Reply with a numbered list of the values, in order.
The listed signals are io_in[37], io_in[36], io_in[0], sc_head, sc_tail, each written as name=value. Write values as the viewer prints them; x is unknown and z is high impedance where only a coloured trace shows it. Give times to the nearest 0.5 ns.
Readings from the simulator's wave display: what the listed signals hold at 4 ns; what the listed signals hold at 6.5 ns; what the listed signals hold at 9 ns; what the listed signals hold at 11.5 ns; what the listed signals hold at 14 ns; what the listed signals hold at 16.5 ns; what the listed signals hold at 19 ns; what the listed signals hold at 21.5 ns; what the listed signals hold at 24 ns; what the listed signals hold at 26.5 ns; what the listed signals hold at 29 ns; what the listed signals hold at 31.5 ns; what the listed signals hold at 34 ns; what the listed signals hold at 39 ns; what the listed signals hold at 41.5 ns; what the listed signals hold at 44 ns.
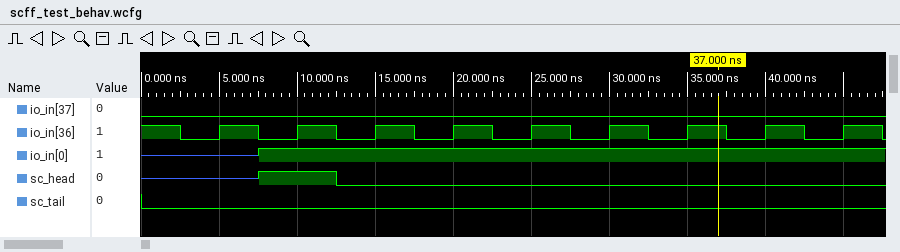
1. io_in[37]=0, io_in[36]=0, io_in[0]=z, sc_head=z, sc_tail=0
2. io_in[37]=0, io_in[36]=1, io_in[0]=z, sc_head=z, sc_tail=0
3. io_in[37]=0, io_in[36]=0, io_in[0]=1, sc_head=1, sc_tail=0
4. io_in[37]=0, io_in[36]=1, io_in[0]=1, sc_head=1, sc_tail=0
5. io_in[37]=0, io_in[36]=0, io_in[0]=1, sc_head=0, sc_tail=0
6. io_in[37]=0, io_in[36]=1, io_in[0]=1, sc_head=0, sc_tail=0
7. io_in[37]=0, io_in[36]=0, io_in[0]=1, sc_head=0, sc_tail=0
8. io_in[37]=0, io_in[36]=1, io_in[0]=1, sc_head=0, sc_tail=0
9. io_in[37]=0, io_in[36]=0, io_in[0]=1, sc_head=0, sc_tail=0
10. io_in[37]=0, io_in[36]=1, io_in[0]=1, sc_head=0, sc_tail=0
11. io_in[37]=0, io_in[36]=0, io_in[0]=1, sc_head=0, sc_tail=0
12. io_in[37]=0, io_in[36]=1, io_in[0]=1, sc_head=0, sc_tail=0
13. io_in[37]=0, io_in[36]=0, io_in[0]=1, sc_head=0, sc_tail=0
14. io_in[37]=0, io_in[36]=0, io_in[0]=1, sc_head=0, sc_tail=0
15. io_in[37]=0, io_in[36]=1, io_in[0]=1, sc_head=0, sc_tail=0
16. io_in[37]=0, io_in[36]=0, io_in[0]=1, sc_head=0, sc_tail=0
